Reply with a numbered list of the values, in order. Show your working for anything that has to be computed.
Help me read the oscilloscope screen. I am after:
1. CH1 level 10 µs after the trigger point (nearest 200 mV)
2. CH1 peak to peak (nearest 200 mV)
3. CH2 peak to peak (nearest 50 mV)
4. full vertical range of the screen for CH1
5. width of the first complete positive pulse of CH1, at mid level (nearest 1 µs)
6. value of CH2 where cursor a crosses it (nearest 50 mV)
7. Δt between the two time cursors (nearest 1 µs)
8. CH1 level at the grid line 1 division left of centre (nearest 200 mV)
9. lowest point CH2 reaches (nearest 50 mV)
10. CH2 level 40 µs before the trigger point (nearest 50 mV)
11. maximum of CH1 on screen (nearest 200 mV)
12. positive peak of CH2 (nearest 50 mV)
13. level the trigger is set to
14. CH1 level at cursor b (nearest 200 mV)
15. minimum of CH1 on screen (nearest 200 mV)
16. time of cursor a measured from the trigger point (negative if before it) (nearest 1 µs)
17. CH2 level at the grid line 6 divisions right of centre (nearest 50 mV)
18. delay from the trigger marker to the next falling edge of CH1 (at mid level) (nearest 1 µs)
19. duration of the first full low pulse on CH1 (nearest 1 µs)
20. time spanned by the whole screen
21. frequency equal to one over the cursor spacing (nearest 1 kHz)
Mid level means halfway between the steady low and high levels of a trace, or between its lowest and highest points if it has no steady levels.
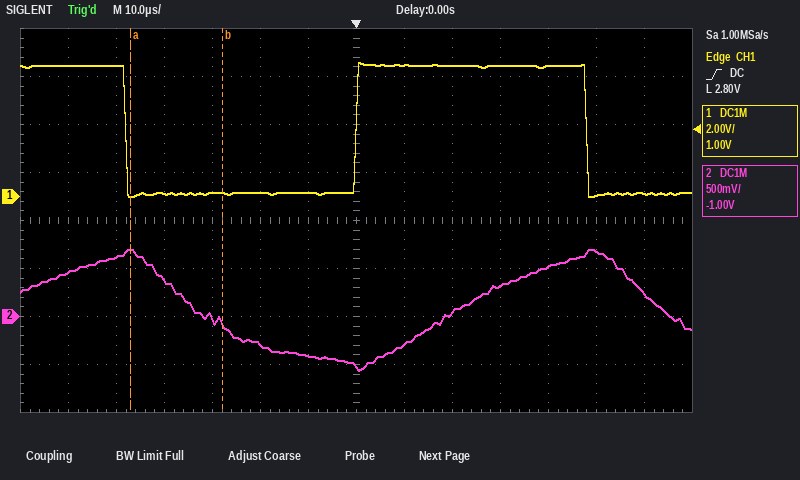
1. 5.4 V
2. 5.6 V − (0.0 V) = 5.6 V
3. 700 mV − (-550 mV) = 1.25 V
4. 16 V
5. 48 µs
6. 700 mV
7. 19 µs
8. 200 mV
9. -550 mV
10. 400 mV
11. 5.6 V
12. 700 mV
13. 2.80 V
14. 200 mV
15. 0.0 V
16. -47 µs
17. 250 mV
18. 48 µs
19. 48 µs
20. 140 µs
21. 1 / 19 µs ≈ 53 kHz
